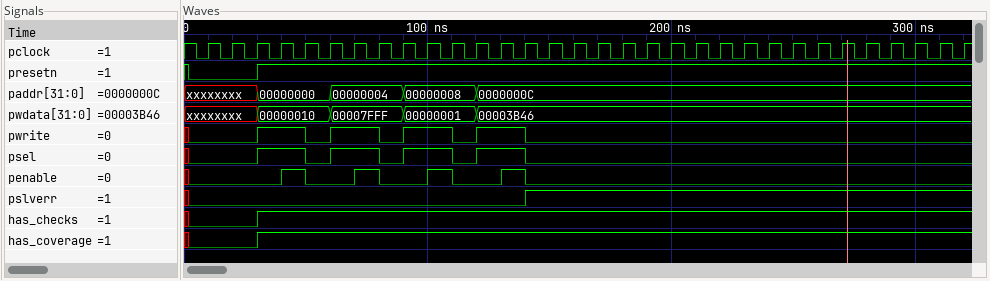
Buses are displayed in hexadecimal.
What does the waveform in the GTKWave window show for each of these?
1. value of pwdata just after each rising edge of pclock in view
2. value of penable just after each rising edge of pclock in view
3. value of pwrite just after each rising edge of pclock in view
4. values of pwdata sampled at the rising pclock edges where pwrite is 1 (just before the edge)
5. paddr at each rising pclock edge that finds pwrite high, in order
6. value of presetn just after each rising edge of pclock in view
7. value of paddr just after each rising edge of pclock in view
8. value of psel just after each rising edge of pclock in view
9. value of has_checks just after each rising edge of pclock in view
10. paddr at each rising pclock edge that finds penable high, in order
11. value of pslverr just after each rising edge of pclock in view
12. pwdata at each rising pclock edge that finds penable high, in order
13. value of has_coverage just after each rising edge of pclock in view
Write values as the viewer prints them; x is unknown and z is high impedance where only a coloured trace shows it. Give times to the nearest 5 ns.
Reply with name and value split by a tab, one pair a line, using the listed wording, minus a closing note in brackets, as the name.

value of pwdata just after each rising edge of pclock in view	xxxxxxxx, xxxxxxxx, 00000010, 00000010, 00000010, 00007FFF, 00007FFF, 00007FFF, 00000001, 00000001, 00000001, 00003B46, 00003B46, 00003B46, 00003B46, 00003B46, 00003B46, 00003B46, 00003B46, 00003B46, 00003B46, 00003B46, 00003B46, 00003B46, 00003B46, 00003B46, 00003B46, 00003B46, 00003B46, 00003B46, 00003B46, 00003B46
value of penable just after each rising edge of pclock in view	0 0 0 1 0 0 1 0 0 1 0 0 1 0 0 0 0 0 0 0 0 0 0 0 0 0 0 0 0 0 0 0
value of pwrite just after each rising edge of pclock in view	0 0 1 1 0 1 1 0 1 1 0 1 1 0 0 0 0 0 0 0 0 0 0 0 0 0 0 0 0 0 0 0
values of pwdata sampled at the rising pclock edges where pwrite is 1	00000010, 00000010, 00007FFF, 00007FFF, 00000001, 00000001, 00003B46, 00003B46
paddr at each rising pclock edge that finds pwrite high, in order	00000000, 00000000, 00000004, 00000004, 00000008, 00000008, 0000000C, 0000000C
value of presetn just after each rising edge of pclock in view	0 0 1 1 1 1 1 1 1 1 1 1 1 1 1 1 1 1 1 1 1 1 1 1 1 1 1 1 1 1 1 1
value of paddr just after each rising edge of pclock in view	xxxxxxxx, xxxxxxxx, 00000000, 00000000, 00000000, 00000004, 00000004, 00000004, 00000008, 00000008, 00000008, 0000000C, 0000000C, 0000000C, 0000000C, 0000000C, 0000000C, 0000000C, 0000000C, 0000000C, 0000000C, 0000000C, 0000000C, 0000000C, 0000000C, 0000000C, 0000000C, 0000000C, 0000000C, 0000000C, 0000000C, 0000000C
value of psel just after each rising edge of pclock in view	0 0 1 1 0 1 1 0 1 1 0 1 1 0 0 0 0 0 0 0 0 0 0 0 0 0 0 0 0 0 0 0
value of has_checks just after each rising edge of pclock in view	0 0 1 1 1 1 1 1 1 1 1 1 1 1 1 1 1 1 1 1 1 1 1 1 1 1 1 1 1 1 1 1
paddr at each rising pclock edge that finds penable high, in order	00000000, 00000004, 00000008, 0000000C
value of pslverr just after each rising edge of pclock in view	0 0 0 0 0 0 0 0 0 0 0 0 0 1 1 1 1 1 1 1 1 1 1 1 1 1 1 1 1 1 1 1
pwdata at each rising pclock edge that finds penable high, in order	00000010, 00007FFF, 00000001, 00003B46
value of has_coverage just after each rising edge of pclock in view	0 0 1 1 1 1 1 1 1 1 1 1 1 1 1 1 1 1 1 1 1 1 1 1 1 1 1 1 1 1 1 1
